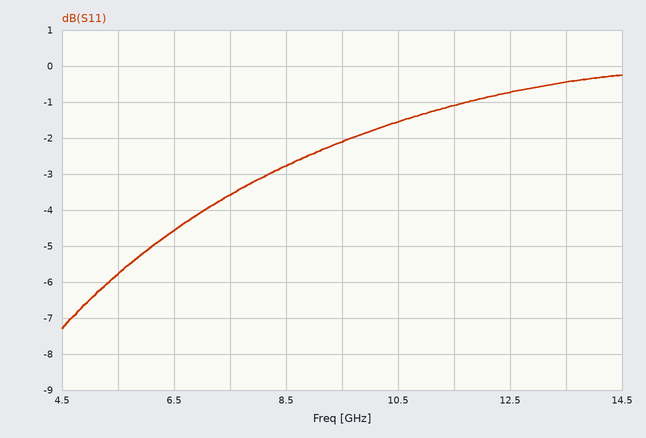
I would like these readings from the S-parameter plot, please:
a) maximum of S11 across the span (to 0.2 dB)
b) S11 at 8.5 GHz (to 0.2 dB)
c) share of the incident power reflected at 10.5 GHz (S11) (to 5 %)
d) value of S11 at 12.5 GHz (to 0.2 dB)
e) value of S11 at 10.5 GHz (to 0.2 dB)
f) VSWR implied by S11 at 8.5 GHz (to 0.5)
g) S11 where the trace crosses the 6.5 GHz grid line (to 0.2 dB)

-0.2 dB
-2.8 dB
70 %
-0.8 dB
-1.6 dB
6.5
-4.6 dB
